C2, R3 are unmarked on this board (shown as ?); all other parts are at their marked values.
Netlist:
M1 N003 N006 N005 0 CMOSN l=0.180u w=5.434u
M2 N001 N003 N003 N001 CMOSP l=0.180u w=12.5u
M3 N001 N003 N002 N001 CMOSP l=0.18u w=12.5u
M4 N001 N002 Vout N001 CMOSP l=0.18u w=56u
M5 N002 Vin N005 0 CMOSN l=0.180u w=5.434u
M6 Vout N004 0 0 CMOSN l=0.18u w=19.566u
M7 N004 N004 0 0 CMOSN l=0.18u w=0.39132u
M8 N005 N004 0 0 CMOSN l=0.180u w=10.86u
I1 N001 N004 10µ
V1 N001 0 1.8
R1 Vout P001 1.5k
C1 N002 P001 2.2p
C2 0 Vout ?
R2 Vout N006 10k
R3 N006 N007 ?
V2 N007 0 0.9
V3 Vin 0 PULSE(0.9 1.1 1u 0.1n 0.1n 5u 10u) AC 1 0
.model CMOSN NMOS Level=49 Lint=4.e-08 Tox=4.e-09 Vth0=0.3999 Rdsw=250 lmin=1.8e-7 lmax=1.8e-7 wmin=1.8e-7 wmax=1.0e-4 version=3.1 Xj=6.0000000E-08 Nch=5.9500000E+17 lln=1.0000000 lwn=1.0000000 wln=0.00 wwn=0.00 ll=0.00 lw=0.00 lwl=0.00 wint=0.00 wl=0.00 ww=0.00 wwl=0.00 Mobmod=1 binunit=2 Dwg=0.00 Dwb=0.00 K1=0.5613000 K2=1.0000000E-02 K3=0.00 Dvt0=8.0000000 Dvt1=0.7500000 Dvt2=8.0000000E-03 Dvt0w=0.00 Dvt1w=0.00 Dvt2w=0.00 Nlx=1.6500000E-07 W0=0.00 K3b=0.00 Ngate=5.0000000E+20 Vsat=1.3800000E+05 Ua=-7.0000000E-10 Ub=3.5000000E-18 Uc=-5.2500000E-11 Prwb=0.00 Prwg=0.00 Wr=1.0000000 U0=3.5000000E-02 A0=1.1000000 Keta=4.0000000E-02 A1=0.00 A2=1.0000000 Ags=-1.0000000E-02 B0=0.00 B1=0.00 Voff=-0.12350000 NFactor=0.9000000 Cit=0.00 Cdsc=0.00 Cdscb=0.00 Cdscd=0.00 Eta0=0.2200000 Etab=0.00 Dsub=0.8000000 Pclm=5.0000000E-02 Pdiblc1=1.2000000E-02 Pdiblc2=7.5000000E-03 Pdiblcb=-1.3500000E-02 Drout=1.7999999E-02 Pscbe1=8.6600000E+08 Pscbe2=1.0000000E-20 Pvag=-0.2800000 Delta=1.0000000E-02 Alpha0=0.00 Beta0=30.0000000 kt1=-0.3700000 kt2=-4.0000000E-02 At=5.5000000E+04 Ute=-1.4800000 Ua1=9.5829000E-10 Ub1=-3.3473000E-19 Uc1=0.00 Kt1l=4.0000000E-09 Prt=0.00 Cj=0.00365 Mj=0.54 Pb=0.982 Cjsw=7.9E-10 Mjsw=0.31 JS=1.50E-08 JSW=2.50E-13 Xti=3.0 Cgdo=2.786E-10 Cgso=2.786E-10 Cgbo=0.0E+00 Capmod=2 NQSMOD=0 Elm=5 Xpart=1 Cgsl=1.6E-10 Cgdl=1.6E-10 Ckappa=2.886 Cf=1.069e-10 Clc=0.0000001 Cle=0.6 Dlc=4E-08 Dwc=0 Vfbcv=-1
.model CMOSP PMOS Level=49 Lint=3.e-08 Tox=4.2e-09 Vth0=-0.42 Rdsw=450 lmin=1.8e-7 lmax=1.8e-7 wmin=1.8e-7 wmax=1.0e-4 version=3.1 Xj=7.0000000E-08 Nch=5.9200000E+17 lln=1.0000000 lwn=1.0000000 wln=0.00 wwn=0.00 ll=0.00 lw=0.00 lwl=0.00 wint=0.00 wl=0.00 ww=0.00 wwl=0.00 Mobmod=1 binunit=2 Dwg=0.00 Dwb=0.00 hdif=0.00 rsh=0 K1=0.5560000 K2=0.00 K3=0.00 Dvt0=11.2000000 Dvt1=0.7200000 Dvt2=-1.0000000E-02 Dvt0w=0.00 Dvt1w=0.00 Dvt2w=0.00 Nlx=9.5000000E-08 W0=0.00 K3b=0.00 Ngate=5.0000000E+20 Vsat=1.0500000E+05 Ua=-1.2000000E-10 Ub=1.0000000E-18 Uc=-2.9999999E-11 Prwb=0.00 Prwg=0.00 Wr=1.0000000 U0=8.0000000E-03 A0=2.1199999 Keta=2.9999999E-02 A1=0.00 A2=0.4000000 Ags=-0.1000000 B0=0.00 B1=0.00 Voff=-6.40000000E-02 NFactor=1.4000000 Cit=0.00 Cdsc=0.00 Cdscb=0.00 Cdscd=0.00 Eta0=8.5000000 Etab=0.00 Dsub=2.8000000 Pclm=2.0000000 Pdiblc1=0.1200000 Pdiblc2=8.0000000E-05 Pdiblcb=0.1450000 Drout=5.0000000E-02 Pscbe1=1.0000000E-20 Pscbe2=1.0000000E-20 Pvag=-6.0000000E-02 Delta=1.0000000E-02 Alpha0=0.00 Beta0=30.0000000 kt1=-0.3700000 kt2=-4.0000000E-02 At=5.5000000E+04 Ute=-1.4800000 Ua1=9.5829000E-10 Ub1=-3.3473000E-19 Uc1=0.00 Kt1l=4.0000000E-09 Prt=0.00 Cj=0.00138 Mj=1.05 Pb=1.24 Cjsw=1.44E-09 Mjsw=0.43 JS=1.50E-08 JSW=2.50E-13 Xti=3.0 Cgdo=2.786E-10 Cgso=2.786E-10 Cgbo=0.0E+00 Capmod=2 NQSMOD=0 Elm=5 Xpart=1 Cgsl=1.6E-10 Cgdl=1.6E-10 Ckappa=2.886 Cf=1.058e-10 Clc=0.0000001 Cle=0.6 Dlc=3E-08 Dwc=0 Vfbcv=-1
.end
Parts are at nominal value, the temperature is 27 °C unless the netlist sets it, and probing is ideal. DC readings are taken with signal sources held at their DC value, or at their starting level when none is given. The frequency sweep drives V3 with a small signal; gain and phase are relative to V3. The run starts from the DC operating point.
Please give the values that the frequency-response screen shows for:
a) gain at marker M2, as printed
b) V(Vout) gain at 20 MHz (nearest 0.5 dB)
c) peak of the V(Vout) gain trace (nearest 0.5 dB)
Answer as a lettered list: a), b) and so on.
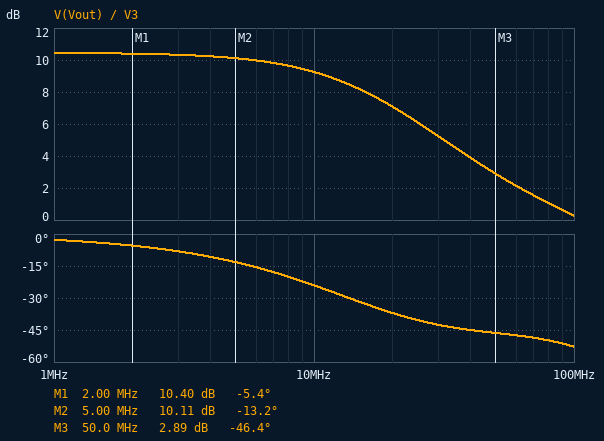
a) 10.11 dB
b) 7.0 dB
c) 10.5 dB
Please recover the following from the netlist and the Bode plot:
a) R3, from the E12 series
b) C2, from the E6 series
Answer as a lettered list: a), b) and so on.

a) 3.9 kΩ
b) 6.8 pF
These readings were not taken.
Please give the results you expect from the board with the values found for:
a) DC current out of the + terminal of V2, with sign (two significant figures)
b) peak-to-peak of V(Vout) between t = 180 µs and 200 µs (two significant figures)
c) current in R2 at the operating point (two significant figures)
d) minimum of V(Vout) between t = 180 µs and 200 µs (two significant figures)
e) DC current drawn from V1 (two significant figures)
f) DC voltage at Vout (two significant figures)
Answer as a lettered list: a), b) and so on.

a) -190 nA
b) 650 mV
c) 190 nA
d) 900 mV
e) 920 µA
f) 900 mV
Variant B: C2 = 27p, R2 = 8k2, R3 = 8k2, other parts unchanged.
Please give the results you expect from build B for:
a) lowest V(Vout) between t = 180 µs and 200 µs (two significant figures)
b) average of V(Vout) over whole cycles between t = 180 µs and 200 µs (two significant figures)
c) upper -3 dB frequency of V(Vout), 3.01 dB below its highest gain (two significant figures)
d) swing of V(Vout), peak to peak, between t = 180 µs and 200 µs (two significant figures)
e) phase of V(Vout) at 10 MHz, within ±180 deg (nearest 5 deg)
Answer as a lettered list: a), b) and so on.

a) 890 mV
b) 1.1 V
c) 32 MHz
d) 400 mV
e) -20 deg
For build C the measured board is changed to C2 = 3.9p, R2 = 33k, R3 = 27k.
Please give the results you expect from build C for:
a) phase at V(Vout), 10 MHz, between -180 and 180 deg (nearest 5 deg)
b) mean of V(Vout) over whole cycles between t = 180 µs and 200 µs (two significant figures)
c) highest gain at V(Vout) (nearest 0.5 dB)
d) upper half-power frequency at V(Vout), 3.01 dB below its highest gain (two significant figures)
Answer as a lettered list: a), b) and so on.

a) -15 deg
b) 1.1 V
c) 6.5 dB
d) 28 MHz
